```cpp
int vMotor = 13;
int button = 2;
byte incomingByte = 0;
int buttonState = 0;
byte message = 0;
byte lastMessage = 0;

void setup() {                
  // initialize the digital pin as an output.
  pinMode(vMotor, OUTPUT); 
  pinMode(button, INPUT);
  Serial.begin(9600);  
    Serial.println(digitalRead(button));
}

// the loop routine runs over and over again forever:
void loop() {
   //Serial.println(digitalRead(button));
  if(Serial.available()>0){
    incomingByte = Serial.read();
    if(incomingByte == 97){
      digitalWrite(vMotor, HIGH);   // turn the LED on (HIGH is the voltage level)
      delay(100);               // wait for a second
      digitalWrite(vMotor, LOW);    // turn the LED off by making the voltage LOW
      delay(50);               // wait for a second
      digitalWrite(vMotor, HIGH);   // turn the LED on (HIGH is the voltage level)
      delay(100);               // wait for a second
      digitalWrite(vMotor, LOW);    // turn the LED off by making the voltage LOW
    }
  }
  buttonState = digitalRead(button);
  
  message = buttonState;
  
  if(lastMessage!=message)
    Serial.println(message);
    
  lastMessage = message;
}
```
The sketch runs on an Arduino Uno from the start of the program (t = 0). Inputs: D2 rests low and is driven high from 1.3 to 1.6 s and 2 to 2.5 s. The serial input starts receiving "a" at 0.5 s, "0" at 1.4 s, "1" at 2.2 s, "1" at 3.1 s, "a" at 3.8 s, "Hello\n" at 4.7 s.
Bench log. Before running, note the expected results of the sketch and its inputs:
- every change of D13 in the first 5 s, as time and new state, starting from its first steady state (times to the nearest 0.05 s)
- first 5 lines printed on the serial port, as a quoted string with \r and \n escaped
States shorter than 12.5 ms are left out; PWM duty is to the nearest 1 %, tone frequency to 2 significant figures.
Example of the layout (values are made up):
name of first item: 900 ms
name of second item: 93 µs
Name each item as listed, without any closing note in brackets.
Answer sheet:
every change of D13 in the first 5 s, as time and new state, starting from its first steady state: 0 s low; 0.5 s high; 0.6 s low; 0.65 s high; 0.75 s low; 3.8 s high; 3.9 s low; 3.95 s high; 4.05 s low
first 5 lines printed on the serial port, as a quoted string with \r and \n escaped: "0\r\n1\r\n0\r\n1\r\n0\r\n"
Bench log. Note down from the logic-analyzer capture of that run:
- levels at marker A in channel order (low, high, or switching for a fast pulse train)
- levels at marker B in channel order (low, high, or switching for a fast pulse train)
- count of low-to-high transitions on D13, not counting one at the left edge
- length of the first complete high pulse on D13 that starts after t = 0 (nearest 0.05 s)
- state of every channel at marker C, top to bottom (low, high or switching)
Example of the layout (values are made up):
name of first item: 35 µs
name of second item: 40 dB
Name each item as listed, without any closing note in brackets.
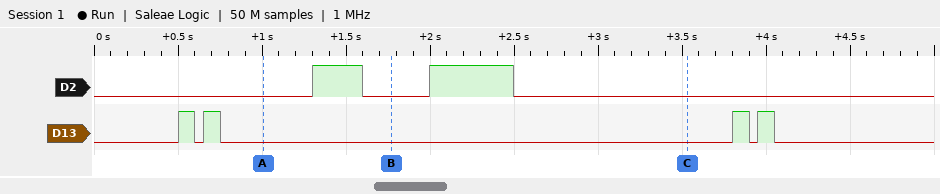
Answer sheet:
levels at marker A in channel order: D2 low, D13 low
levels at marker B in channel order: D2 low, D13 low
count of low-to-high transitions on D13, not counting one at the left edge: 4
length of the first complete high pulse on D13 that starts after t = 0: 0.10 s
state of every channel at marker C, top to bottom: D2 low, D13 low
